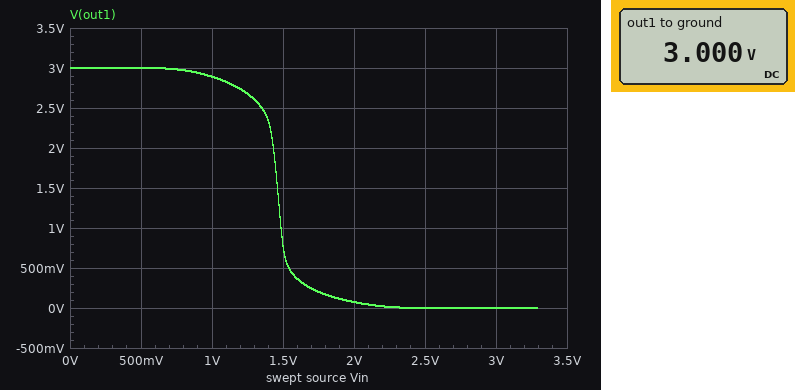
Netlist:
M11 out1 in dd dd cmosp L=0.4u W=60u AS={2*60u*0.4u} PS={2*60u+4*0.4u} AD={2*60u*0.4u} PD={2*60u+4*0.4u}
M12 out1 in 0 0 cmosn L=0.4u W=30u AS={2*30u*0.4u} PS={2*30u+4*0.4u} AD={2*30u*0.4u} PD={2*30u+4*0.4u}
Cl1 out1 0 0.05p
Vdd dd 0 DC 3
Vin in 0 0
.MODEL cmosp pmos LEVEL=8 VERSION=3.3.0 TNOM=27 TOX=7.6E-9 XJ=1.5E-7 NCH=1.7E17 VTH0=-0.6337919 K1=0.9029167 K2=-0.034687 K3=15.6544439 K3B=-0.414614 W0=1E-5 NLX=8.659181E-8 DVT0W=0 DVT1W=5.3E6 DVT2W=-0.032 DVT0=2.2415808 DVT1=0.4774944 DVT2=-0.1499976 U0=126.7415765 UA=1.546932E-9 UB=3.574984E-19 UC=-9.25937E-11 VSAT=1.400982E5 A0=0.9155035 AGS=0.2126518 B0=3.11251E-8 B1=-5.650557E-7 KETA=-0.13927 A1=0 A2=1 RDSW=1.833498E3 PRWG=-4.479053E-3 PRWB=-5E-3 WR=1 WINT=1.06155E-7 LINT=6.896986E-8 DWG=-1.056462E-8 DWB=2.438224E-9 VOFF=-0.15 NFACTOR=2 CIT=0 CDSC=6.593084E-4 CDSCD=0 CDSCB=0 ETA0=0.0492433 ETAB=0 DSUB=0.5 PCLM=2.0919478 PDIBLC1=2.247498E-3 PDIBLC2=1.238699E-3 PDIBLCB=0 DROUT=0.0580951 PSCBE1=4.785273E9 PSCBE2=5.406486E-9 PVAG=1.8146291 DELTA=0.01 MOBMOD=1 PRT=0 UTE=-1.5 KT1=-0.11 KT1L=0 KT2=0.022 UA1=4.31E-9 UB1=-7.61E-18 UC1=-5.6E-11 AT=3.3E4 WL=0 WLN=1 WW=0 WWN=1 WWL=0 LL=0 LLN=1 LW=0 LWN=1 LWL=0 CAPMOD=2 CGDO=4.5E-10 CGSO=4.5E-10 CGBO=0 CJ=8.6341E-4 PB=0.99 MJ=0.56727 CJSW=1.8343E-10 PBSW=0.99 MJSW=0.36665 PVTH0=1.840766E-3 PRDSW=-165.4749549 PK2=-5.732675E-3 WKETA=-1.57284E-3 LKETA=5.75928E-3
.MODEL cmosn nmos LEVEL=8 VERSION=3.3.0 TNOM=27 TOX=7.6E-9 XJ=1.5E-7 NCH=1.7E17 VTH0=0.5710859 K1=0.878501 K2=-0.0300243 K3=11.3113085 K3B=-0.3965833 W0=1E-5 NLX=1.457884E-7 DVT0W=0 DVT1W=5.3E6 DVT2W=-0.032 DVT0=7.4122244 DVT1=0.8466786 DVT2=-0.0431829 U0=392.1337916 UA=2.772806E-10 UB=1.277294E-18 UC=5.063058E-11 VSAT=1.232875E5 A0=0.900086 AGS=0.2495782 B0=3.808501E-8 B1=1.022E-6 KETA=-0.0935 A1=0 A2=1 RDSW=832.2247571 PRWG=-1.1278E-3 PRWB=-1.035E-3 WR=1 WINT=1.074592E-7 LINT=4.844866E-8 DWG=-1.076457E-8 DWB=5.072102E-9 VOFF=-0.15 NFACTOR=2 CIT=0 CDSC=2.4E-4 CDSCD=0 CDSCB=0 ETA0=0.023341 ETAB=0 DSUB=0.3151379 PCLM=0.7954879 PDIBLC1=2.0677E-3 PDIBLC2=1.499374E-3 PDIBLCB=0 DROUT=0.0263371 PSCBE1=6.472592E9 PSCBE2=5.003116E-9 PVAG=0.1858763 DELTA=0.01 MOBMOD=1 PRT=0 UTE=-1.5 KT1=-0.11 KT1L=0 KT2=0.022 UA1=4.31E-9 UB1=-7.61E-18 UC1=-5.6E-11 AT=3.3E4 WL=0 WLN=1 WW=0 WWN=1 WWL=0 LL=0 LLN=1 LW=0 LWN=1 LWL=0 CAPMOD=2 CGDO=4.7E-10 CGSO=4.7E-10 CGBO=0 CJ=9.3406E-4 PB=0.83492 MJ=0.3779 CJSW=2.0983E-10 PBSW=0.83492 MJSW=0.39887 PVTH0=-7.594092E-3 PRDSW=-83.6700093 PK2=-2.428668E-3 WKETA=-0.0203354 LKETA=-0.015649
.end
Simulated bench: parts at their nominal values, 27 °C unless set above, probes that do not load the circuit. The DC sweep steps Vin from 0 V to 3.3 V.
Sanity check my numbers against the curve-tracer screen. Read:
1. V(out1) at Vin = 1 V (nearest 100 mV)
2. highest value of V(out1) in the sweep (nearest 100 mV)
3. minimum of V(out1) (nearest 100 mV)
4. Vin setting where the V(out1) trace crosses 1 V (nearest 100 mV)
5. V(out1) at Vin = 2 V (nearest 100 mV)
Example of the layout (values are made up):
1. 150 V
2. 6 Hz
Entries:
1. 2.9 V
2. 3.0 V
3. 0 V
4. 1.5 V
5. 100 mV
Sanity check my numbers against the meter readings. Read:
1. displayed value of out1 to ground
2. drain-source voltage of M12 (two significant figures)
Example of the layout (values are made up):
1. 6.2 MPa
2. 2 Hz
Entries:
1. 3.000 V
2. 3.0 V
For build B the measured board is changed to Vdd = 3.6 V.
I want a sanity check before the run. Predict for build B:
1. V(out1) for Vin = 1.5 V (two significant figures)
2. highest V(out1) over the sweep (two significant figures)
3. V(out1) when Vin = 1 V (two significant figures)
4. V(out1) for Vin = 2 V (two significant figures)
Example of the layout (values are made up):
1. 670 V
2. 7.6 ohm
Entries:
1. 3.1 V
2. 3.6 V
3. 3.5 V
4. 400 mV
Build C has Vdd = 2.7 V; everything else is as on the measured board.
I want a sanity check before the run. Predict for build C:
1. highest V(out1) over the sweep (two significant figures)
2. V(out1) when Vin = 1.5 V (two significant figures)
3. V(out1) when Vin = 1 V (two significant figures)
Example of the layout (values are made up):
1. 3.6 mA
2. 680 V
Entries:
1. 2.7 V
2. 220 mV
3. 2.6 V
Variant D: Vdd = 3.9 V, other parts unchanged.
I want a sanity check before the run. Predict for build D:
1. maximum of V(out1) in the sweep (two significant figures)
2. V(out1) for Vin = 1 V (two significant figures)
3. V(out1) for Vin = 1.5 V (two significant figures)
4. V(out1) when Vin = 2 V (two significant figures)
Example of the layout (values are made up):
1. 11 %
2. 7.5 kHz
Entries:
1. 3.9 V
2. 3.8 V
3. 3.5 V
4. 790 mV
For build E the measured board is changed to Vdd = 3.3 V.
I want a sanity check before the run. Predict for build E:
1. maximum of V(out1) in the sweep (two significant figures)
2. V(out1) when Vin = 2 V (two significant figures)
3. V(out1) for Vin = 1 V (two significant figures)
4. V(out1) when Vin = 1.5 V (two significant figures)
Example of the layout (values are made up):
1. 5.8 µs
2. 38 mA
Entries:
1. 3.3 V
2. 200 mV
3. 3.2 V
4. 2.7 V
